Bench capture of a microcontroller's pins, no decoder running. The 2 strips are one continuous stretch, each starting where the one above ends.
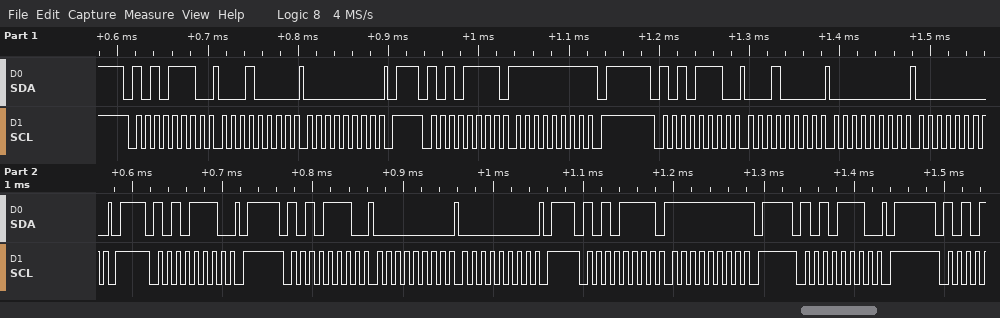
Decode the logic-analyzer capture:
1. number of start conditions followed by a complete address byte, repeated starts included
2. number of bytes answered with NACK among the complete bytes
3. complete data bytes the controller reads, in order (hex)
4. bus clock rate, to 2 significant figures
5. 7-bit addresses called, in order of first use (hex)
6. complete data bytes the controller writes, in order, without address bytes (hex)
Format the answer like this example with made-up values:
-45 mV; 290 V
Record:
7; 2; FF FF; 100 kHz; 0x57; 10 00 10 00 00 00 00
